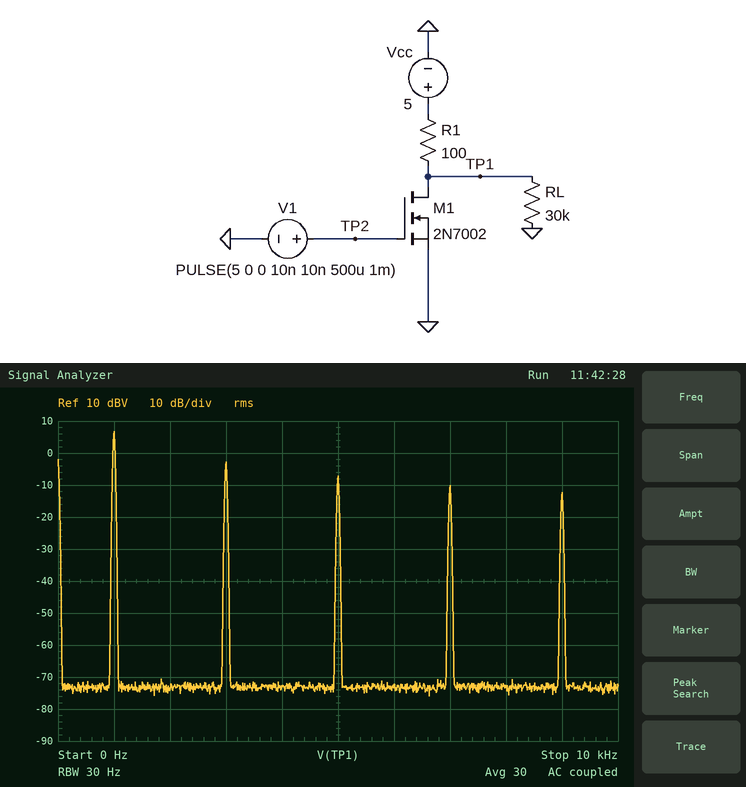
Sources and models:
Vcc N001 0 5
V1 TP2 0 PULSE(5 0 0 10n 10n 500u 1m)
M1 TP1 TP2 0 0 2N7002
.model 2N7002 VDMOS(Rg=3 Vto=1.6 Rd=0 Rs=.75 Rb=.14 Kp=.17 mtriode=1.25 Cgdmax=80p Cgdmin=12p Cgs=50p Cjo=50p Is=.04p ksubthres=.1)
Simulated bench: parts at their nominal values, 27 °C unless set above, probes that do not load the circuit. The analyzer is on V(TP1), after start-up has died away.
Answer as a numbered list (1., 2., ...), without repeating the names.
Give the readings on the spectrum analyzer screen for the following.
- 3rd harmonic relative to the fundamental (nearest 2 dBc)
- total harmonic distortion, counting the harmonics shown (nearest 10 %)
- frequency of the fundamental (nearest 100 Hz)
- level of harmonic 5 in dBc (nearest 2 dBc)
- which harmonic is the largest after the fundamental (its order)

1. -10 dBc
2. 40 %
3. 1.0 kHz
4. -14 dBc
5. 3
